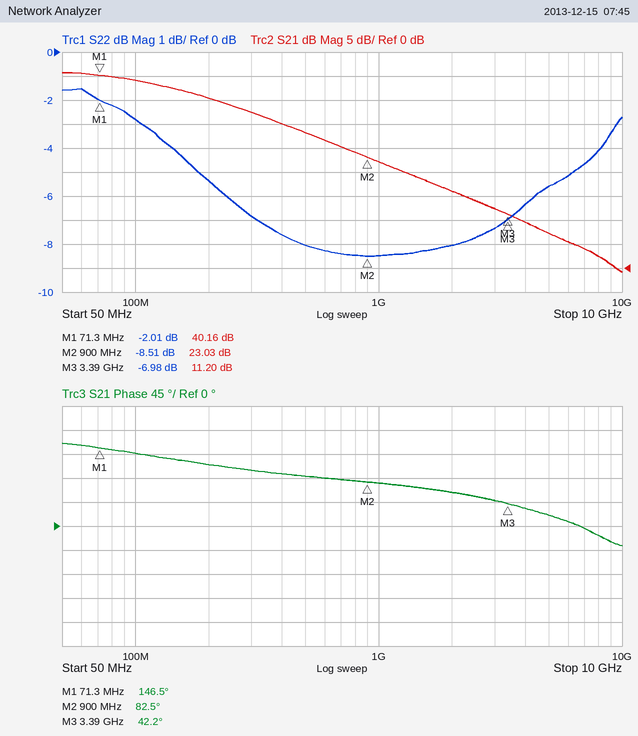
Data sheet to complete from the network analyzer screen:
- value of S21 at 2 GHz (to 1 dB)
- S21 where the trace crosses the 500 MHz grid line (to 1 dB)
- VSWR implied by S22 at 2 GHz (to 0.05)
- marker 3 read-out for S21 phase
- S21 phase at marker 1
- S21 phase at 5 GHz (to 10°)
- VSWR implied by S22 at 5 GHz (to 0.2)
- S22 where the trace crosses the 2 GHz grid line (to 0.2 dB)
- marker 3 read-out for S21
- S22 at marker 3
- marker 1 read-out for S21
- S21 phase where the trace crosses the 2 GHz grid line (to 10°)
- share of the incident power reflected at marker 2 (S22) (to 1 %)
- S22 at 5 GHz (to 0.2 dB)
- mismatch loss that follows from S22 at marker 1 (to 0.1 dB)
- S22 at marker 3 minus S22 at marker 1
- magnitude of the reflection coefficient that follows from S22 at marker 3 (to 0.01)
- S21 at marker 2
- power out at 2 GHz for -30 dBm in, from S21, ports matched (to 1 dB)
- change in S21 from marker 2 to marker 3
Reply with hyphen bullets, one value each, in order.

- 16 dB
- 28 dB
- 2.30
- 42.2°
- 146.5°
- 20°
- 3.2
- -8.0 dB
- 11.20 dB
- -6.98 dB
- 40.16 dB
- 60°
- 14 %
- -5.6 dB
- 4.3 dB
- -4.97 dB
- 0.45
- 23.03 dB
- -14 dBm
- -11.83 dB
